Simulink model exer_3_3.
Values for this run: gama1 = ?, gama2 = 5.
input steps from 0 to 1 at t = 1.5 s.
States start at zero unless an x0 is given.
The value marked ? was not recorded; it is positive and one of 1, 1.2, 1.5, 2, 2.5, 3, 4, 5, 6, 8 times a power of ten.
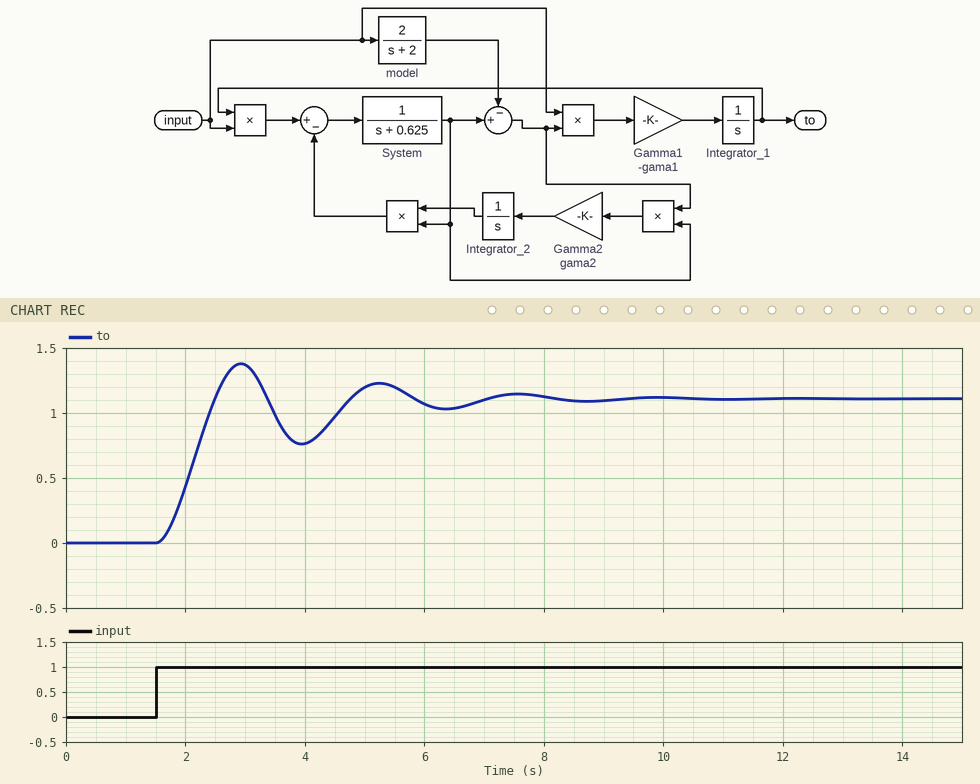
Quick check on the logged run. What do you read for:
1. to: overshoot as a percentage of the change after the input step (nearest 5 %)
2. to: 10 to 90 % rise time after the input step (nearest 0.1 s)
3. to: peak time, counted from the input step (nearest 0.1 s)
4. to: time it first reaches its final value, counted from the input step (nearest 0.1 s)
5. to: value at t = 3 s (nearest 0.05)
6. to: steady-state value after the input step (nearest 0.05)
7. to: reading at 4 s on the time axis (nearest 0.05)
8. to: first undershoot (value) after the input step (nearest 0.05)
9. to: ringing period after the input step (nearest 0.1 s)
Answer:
25 %
0.7 s
1.4 s
1.0 s
1.35
1.10
0.75
0.75
2.3 s
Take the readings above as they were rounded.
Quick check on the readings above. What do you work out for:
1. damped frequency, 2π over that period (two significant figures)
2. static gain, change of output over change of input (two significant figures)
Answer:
2.7 rad/s
1.1
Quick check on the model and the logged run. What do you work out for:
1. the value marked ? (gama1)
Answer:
2.5
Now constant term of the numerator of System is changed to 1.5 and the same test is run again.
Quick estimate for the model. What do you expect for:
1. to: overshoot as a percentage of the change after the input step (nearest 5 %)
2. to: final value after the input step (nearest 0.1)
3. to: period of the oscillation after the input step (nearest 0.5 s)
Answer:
25 %
0.8
2.0 s
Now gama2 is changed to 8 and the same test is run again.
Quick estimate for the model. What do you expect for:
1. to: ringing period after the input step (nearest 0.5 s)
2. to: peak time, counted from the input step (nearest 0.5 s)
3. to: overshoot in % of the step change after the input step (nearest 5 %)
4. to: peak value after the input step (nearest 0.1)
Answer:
2.0 s
1.5 s
15 %
1.3
